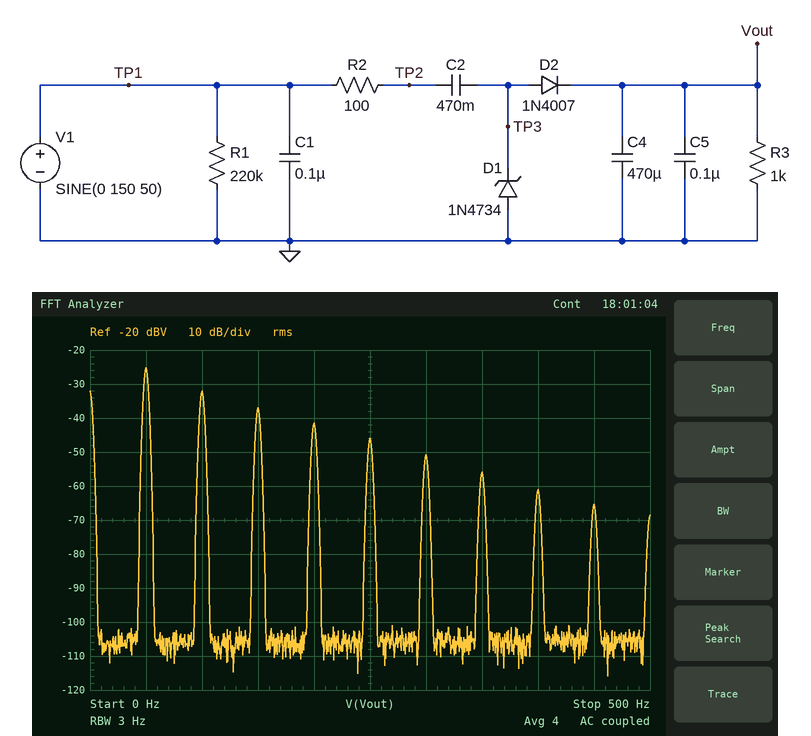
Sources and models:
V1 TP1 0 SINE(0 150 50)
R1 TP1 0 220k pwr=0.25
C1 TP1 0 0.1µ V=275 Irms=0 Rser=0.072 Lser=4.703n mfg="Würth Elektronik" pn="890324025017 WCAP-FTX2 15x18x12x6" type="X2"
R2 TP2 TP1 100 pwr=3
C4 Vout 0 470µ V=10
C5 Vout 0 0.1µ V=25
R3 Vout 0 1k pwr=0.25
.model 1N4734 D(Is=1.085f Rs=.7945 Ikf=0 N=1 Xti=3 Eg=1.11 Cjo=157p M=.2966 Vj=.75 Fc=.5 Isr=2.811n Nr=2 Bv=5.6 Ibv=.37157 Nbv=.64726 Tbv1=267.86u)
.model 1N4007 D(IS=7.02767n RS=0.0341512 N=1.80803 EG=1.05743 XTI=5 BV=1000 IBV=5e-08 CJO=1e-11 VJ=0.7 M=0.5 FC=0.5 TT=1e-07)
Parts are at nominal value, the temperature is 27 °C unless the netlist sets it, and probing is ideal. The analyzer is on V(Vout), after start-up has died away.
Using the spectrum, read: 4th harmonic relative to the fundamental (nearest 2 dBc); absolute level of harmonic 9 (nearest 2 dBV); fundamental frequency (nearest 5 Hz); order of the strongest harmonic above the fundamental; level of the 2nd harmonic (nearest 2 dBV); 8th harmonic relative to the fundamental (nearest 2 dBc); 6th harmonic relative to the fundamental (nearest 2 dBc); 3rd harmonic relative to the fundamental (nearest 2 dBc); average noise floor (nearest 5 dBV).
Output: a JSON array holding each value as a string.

["-16 dBc", "-66 dBV", "50 Hz", "2", "-32 dBV", "-36 dBc", "-26 dBc", "-12 dBc", "-105 dBV"]
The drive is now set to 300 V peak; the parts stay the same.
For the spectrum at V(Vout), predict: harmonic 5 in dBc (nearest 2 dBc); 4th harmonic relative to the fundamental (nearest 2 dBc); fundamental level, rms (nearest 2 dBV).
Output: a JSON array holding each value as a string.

["-18 dBc", "-14 dBc", "-24 dBV"]
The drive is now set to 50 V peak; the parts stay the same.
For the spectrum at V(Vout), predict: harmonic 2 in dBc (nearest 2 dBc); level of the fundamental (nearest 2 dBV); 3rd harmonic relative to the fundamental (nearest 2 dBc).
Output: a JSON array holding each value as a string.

["-8 dBc", "-26 dBV", "-16 dBc"]
